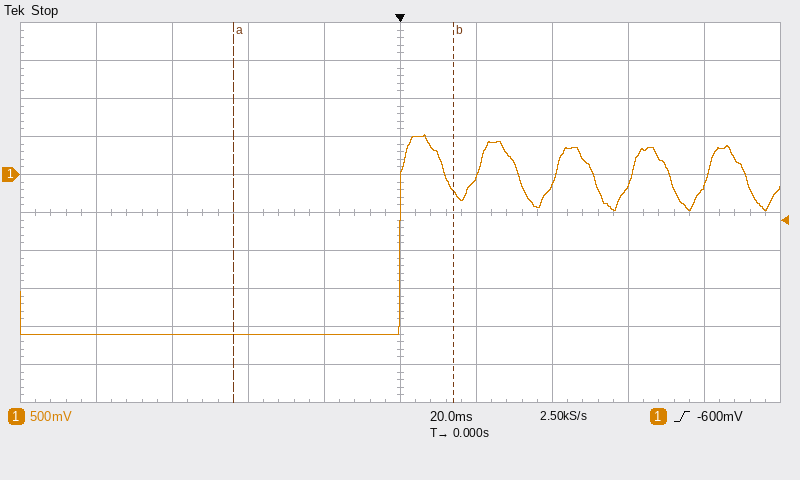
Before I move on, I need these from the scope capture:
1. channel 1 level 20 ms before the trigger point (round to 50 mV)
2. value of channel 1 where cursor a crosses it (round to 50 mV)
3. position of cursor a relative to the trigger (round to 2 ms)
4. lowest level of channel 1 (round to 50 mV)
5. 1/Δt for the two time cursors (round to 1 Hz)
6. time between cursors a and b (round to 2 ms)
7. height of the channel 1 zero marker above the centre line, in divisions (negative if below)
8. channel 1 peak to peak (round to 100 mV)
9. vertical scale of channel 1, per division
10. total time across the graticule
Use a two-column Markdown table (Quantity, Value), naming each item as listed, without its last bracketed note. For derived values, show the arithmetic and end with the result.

| Quantity | Value |
|---|---|
| channel 1 level 20 ms before the trigger point | -2.10 V |
| value of channel 1 where cursor a crosses it | -2.10 V |
| position of cursor a relative to the trigger | -44 ms |
| lowest level of channel 1 | -2.10 V |
| 1/Δt for the two time cursors | 1 / 58 ms ≈ 17 Hz |
| time between cursors a and b | 58 ms |
| height of the channel 1 zero marker above the centre line, in divisions | +1.0 div |
| channel 1 peak to peak | 2.60 V |
| vertical scale of channel 1, per division | 500 mV |
| total time across the graticule | 200 ms |
